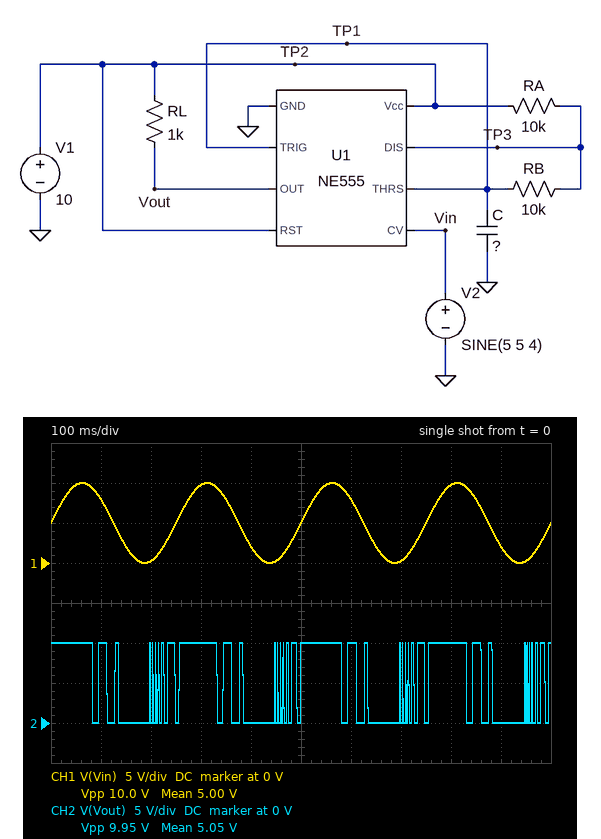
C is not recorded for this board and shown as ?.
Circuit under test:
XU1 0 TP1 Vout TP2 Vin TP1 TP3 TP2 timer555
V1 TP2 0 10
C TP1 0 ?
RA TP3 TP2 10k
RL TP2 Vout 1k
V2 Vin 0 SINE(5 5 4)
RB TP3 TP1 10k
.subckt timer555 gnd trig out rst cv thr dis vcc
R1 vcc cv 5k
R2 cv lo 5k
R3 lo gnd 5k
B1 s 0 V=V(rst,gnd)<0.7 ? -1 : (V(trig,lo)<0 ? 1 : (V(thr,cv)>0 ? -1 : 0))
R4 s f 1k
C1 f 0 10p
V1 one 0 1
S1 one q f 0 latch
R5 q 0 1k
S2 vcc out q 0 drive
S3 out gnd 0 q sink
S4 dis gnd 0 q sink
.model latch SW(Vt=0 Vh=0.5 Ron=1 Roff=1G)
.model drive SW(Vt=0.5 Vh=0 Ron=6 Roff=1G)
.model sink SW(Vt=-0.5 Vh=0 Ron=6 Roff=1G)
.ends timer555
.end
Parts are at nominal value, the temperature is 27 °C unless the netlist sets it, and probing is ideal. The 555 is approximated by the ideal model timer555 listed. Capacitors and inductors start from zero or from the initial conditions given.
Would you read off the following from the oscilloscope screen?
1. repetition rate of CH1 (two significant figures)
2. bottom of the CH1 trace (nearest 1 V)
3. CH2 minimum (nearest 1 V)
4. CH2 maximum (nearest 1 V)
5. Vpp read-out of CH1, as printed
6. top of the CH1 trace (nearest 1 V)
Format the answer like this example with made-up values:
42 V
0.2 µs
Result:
4.0 Hz
0 V
0 V
10 V
10.0 V
10 V
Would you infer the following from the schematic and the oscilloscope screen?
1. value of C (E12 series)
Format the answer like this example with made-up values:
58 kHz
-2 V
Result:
1.5 µF
